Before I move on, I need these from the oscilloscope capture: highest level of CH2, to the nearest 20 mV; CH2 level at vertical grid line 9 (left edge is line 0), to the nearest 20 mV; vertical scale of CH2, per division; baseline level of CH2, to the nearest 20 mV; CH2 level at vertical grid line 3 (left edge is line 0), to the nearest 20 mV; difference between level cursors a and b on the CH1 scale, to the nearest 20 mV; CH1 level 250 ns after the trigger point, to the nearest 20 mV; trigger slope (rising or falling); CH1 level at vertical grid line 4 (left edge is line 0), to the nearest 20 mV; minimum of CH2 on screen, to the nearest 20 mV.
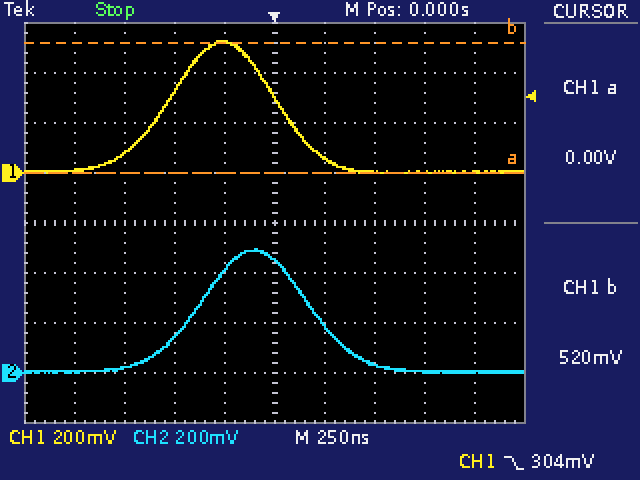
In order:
500 mV
0 mV
200 mV
0 mV
140 mV
520 mV
60 mV
falling
520 mV
0 mV
